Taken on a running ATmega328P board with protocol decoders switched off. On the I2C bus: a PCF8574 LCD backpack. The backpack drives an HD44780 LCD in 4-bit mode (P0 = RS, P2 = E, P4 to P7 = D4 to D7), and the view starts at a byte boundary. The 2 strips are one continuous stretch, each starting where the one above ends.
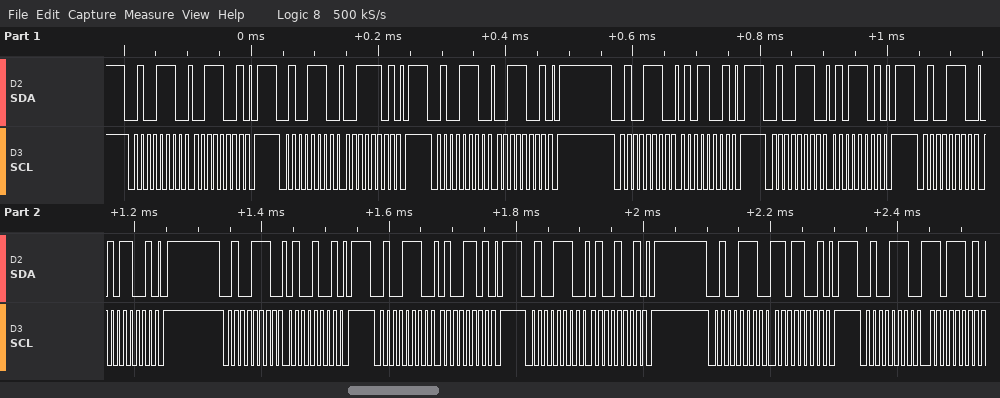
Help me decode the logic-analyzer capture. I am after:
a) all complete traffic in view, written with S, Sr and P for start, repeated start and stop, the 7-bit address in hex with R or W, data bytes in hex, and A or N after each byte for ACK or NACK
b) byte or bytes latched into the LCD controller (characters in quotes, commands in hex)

S 27W A 39 A P S 27W A 3D A P S 27W A 39 A P S 27W A 59 A P S 27W A 5D A P S 27W A 59 A P S 27W A 49 A P S 27W A 4D A P S 27W A 49 A P S 27W A D9 A P S 27W A DD A
'5'
